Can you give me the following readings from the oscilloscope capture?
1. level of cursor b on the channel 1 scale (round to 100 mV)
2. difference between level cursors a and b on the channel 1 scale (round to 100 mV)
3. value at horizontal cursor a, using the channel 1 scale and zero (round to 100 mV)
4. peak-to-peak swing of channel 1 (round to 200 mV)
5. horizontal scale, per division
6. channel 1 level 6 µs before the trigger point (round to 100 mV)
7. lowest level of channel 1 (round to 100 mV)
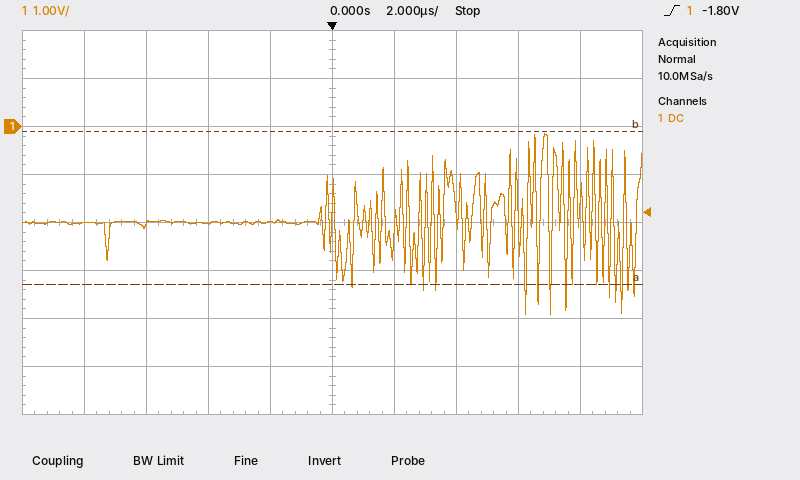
-100 mV
3.2 V
-3.3 V
3.8 V
2 µs
-2.0 V
-3.9 V
